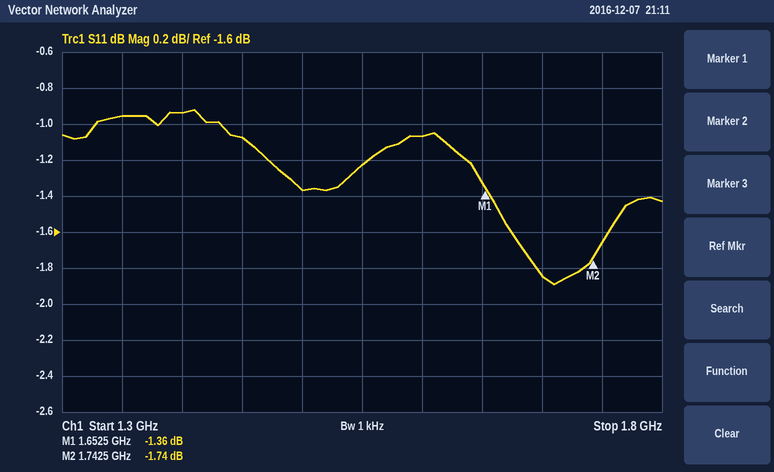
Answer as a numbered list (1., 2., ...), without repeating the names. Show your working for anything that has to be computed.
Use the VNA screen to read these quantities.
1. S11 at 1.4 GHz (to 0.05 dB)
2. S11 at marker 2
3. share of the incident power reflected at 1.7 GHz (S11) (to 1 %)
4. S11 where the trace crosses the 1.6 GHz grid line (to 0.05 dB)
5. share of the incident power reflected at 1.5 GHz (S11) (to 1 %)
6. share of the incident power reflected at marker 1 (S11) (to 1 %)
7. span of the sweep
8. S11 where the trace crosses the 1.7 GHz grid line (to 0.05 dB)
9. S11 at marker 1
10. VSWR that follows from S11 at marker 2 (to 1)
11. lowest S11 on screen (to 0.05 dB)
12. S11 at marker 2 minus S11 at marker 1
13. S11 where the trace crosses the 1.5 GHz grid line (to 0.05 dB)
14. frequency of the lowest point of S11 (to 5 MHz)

1. -0.95 dB
2. -1.74 dB
3. 10^(-1.85/10) ≈ 65 %
4. -1.05 dB
5. 10^(-1.35/10) ≈ 73 %
6. 10^(-1.36/10) ≈ 73 %
7. 500 MHz
8. -1.85 dB
9. -1.36 dB
10. (1 + 0.8185)/(1 − 0.8185) ≈ 10
11. -1.90 dB
12. -1.74 − (-1.36) = -0.38 dB
13. -1.35 dB
14. 1.710 GHz
